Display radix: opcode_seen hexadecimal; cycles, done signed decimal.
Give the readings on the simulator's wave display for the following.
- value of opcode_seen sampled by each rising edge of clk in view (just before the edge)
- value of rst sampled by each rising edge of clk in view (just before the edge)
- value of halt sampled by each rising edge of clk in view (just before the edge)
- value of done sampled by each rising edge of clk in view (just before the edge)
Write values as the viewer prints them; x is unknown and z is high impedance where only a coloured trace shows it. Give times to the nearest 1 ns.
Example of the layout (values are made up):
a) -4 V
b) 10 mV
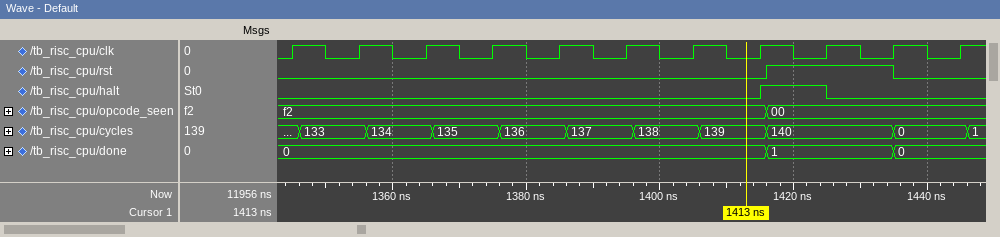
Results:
a) f2, f2, f2, f2, f2, f2, f2, f2, 00, 00, 00
b) 0 0 0 0 0 0 0 0 1 1 0
c) 0 0 0 0 0 0 0 0 1 0 0
d) 0, 0, 0, 0, 0, 0, 0, 0, 1, 1, 0
